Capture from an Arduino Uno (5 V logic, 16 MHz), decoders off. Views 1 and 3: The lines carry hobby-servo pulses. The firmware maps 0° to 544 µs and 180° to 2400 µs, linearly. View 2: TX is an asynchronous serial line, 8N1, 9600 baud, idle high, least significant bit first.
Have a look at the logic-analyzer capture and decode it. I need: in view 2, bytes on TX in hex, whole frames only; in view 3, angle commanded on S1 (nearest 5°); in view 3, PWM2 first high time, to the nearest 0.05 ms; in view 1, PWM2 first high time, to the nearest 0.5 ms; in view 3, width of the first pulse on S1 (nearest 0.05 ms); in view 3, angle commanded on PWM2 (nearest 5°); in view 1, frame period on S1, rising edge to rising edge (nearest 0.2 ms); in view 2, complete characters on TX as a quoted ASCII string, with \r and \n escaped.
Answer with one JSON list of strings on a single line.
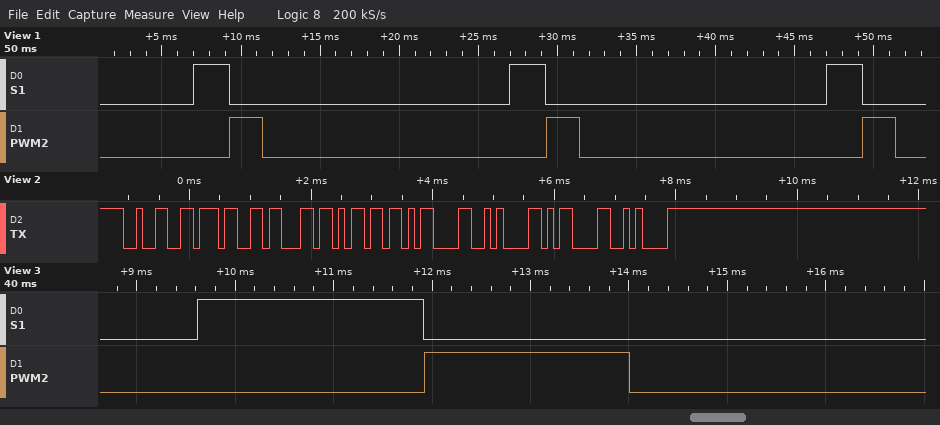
["32 37 63 6D 0D 0A 0D 0A", "170°", "2.10 ms", "2.0 ms", "2.30 ms", "150°", "20.0 ms", "\"27cm\\r\\n\\r\\n\""]
